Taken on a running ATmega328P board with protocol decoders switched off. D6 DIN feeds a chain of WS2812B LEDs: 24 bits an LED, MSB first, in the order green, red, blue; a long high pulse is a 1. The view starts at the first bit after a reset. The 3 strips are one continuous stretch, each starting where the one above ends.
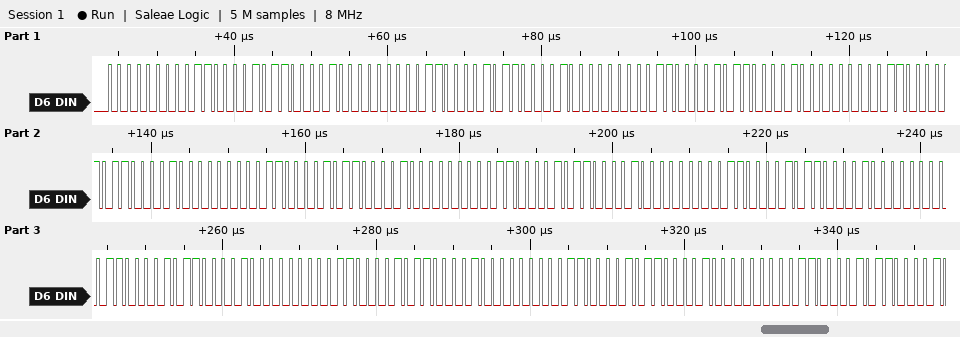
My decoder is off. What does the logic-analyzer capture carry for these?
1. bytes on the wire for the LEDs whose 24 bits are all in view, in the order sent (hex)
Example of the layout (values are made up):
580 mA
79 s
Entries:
00 61 61 00 61 61 00 61 61 00 61 61 00 61 61 00 61 61 00 61 61 00 61 61 00 61 61 00 61 61 00 61 61
